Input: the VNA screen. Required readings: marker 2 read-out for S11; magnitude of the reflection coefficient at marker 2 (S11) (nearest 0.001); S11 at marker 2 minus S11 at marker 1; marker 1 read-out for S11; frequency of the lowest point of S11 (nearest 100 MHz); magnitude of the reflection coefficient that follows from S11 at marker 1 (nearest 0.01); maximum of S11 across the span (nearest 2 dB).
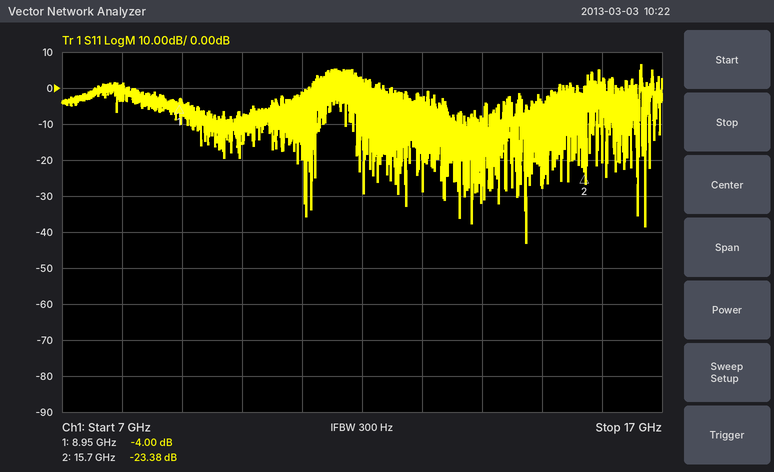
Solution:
-23.38 dB
0.068
-19.38 dB
-4.00 dB
14.7 GHz
0.63
6 dB
